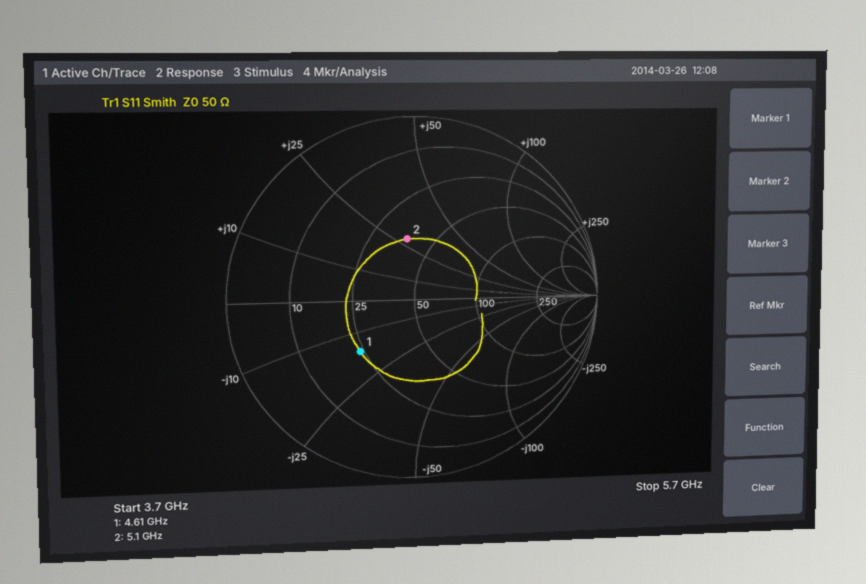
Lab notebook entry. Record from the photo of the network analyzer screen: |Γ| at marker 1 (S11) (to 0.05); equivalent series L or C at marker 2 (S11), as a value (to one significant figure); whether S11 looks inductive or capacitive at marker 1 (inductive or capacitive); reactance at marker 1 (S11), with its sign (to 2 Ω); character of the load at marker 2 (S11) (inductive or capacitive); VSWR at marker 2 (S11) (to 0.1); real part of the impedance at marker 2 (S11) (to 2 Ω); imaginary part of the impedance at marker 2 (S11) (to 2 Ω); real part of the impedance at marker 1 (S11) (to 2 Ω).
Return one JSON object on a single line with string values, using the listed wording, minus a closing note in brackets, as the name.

{"|Γ| at marker 1 (S11)": "0.40", "equivalent series L or C at marker 2 (S11), as a value": "900 pH", "whether S11 looks inductive or capacitive at marker 1": "capacitive", "reactance at marker 1 (S11), with its sign": "-16 Ω", "character of the load at marker 2 (S11)": "inductive", "VSWR at marker 2 (S11)": "2.0", "real part of the impedance at marker 2 (S11)": "38 Ω", "imaginary part of the impedance at marker 2 (S11)": "+28 Ω", "real part of the impedance at marker 1 (S11)": "24 Ω"}
